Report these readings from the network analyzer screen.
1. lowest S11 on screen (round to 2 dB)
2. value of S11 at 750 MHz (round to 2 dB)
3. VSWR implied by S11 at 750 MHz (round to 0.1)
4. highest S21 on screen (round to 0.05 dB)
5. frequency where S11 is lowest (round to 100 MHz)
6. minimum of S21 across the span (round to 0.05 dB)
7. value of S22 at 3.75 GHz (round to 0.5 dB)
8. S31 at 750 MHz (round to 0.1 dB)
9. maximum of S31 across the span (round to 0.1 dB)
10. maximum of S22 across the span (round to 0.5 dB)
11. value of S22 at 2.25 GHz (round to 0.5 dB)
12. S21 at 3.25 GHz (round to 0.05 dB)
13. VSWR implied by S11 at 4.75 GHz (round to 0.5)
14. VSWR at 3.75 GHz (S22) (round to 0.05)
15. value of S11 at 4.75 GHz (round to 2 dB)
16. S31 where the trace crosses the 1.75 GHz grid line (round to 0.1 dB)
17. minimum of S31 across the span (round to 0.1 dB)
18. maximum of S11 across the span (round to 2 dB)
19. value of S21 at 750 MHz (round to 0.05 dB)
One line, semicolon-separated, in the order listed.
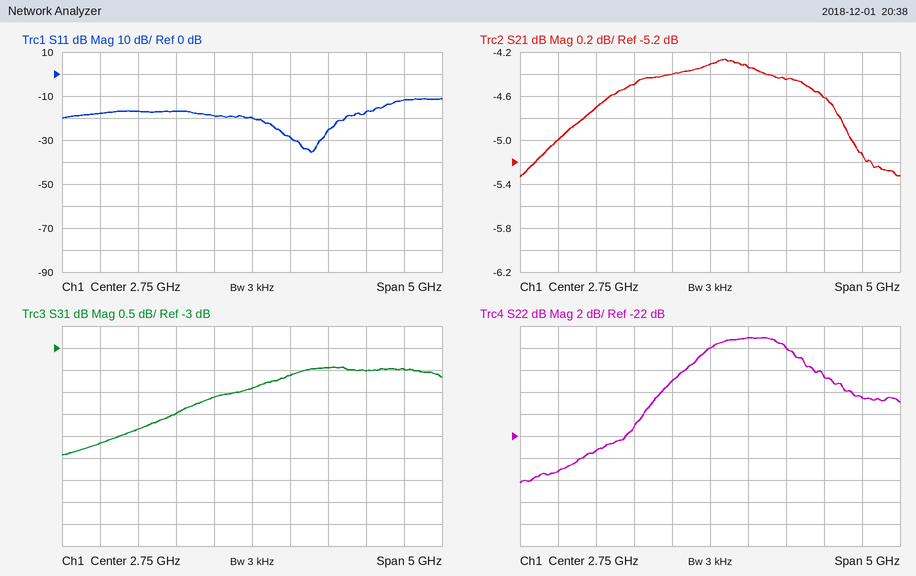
-36 dB; -18 dB; 1.3; -4.25 dB; 3.5 GHz; -5.35 dB; -14.0 dB; -5.2 dB; -3.4 dB; -13.0 dB; -17.0 dB; -4.35 dB; 1.5; 1.50; -12 dB; -4.5 dB; -5.4 dB; -12 dB; -5.00 dB
